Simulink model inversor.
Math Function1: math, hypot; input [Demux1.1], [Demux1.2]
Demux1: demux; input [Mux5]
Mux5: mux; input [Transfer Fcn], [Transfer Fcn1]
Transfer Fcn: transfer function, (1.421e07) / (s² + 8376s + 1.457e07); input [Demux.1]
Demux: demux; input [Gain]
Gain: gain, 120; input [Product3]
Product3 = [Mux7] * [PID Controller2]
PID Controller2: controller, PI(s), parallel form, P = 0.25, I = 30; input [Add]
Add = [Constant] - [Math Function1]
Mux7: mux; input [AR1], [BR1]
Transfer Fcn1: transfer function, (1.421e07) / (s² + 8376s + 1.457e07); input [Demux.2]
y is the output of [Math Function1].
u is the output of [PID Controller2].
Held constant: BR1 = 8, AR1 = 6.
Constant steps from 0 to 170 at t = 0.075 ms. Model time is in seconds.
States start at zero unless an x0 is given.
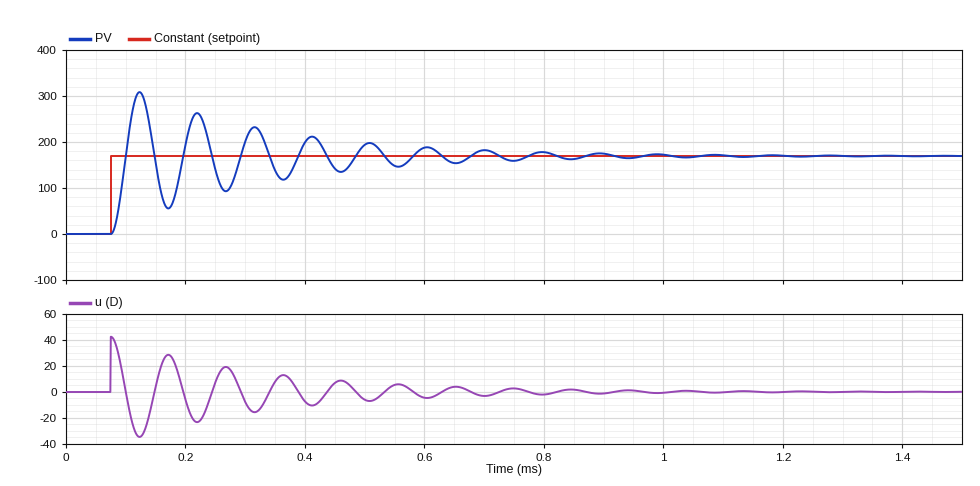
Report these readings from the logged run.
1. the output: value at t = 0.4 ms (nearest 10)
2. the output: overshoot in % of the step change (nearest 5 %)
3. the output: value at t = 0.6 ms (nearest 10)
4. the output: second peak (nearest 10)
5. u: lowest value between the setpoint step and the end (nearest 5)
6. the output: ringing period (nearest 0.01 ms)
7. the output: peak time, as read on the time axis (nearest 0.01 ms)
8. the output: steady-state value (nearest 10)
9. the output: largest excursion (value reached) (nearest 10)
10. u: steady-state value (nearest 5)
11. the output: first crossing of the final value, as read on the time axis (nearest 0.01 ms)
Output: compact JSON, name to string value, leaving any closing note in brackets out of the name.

{"the output: value at t = 0.4 ms": "200", "the output: overshoot in % of the step change": "80 %", "the output: value at t = 0.6 ms": "190", "the output: second peak": "260", "u: lowest value between the setpoint step and the end": "-35", "the output: ringing period": "0.10 ms", "the output: peak time, as read on the time axis": "0.12 ms", "the output: steady-state value": "170", "the output: largest excursion (value reached)": "310", "u: steady-state value": "0", "the output: first crossing of the final value, as read on the time axis": "0.10 ms"}
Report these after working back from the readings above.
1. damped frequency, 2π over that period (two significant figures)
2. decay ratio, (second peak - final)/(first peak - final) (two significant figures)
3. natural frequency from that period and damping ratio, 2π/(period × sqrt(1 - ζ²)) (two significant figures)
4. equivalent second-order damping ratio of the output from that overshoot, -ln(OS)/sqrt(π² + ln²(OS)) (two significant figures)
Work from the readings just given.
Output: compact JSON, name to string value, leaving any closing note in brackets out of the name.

{"damped frequency, 2π over that period": "63 rad/ms", "decay ratio, (second peak - final)/(first peak - final)": "0.64", "natural frequency from that period and damping ratio, 2π/(period × sqrt(1 - ζ²))": "63 rad/ms", "equivalent second-order damping ratio of the output from that overshoot, -ln(OS)/sqrt(π² + ln²(OS))": "0.071"}
